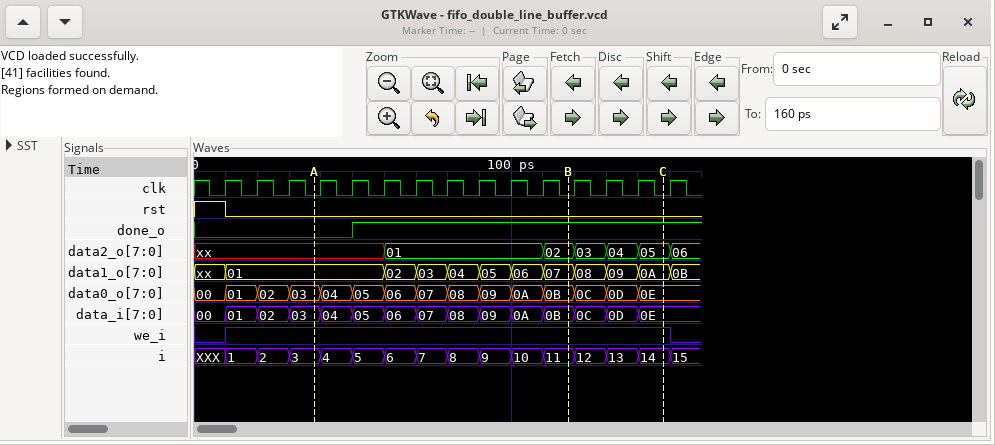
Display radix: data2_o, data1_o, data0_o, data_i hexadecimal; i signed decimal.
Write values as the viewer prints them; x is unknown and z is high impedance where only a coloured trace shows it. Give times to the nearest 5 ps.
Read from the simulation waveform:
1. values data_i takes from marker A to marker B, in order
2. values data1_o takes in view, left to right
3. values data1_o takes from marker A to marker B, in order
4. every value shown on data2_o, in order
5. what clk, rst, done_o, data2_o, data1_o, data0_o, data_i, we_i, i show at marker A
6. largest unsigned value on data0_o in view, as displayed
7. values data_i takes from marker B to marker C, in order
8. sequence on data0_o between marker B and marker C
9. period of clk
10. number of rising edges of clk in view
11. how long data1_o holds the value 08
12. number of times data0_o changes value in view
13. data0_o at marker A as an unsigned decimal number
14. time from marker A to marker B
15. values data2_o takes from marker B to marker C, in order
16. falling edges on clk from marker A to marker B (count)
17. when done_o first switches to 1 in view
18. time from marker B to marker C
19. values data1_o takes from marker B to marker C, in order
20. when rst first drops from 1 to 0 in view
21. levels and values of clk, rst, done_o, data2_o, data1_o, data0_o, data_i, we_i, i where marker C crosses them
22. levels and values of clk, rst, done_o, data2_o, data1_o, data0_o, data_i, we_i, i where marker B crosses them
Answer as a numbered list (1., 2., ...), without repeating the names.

1. 03, 04, 05, 06, 07, 08, 09, 0A, 0B
2. xx, 01, 02, 03, 04, 05, 06, 07, 08, 09, 0A, 0B
3. 01, 02, 03, 04, 05, 06, 07
4. xx, 01, 02, 03, 04, 05, 06
5. clk=0, rst=0, done_o=0, data2_o=xx, data1_o=01, data0_o=03, data_i=03, we_i=1, i=3
6. 0E
7. 0B, 0C, 0D, 0E
8. 0B, 0C, 0D, 0E
9. 10 ps
10. 15
11. 10 ps
12. 14
13. 3
14. 80 ps
15. 02, 03, 04, 05
16. 8
17. 50 ps
18. 30 ps
19. 07, 08, 09, 0A
20. 10 ps
21. clk=0, rst=0, done_o=1, data2_o=05, data1_o=0A, data0_o=0E, data_i=0E, we_i=1, i=14
22. clk=0, rst=0, done_o=1, data2_o=02, data1_o=07, data0_o=0B, data_i=0B, we_i=1, i=11
